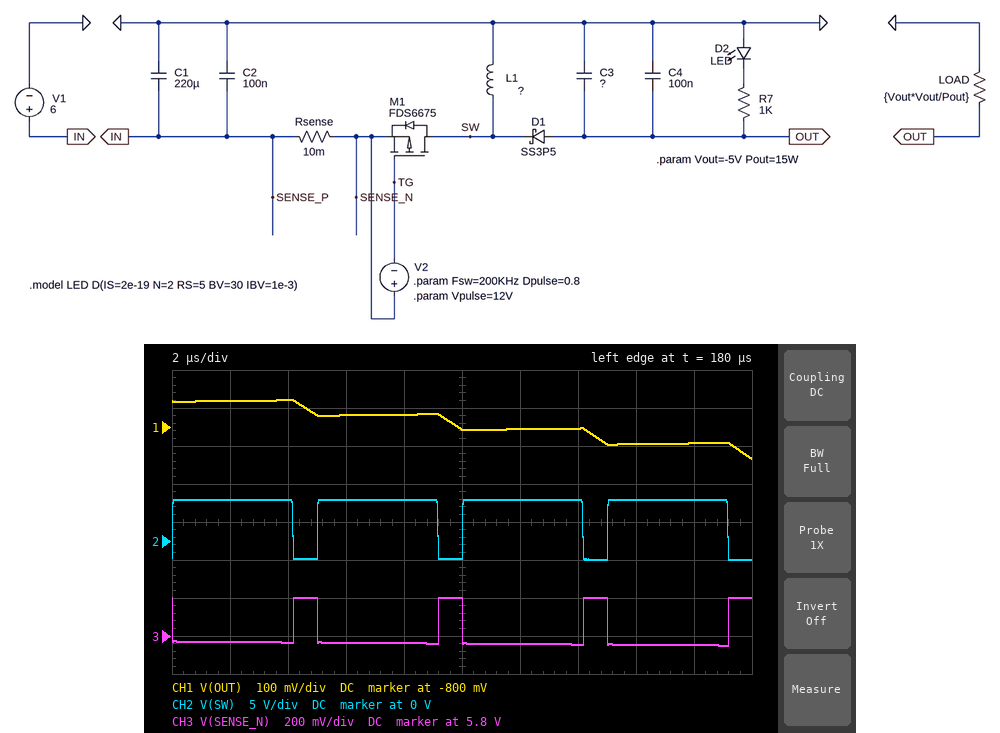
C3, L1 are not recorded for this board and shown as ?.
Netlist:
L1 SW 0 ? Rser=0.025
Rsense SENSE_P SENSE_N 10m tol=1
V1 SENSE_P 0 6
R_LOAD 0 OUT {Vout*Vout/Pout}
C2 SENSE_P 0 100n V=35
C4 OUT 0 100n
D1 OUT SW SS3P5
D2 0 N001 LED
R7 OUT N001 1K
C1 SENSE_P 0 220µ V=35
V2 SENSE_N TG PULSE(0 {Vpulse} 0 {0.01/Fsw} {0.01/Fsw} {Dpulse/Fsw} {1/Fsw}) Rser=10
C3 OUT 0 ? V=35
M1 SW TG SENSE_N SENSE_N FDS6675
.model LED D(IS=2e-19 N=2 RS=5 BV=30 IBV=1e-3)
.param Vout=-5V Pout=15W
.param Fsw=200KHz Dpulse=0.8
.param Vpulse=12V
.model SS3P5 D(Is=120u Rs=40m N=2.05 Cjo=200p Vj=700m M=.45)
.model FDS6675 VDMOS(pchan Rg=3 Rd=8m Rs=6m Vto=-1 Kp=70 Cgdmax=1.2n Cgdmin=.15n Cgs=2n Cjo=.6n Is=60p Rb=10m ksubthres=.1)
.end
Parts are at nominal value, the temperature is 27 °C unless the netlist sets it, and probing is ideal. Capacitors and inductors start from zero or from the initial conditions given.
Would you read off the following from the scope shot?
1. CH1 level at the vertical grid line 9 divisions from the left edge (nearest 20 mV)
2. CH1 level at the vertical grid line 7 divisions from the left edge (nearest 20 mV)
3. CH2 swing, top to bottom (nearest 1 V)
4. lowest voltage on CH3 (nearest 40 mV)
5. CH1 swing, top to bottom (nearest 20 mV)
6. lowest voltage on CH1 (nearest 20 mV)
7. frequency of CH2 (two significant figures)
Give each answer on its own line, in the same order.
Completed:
-840 mV
-800 mV
8 V
5.76 V
160 mV
-880 mV
200 kHz
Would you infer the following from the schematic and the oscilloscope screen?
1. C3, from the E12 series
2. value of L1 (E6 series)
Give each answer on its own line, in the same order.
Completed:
470 µF
33 µH
